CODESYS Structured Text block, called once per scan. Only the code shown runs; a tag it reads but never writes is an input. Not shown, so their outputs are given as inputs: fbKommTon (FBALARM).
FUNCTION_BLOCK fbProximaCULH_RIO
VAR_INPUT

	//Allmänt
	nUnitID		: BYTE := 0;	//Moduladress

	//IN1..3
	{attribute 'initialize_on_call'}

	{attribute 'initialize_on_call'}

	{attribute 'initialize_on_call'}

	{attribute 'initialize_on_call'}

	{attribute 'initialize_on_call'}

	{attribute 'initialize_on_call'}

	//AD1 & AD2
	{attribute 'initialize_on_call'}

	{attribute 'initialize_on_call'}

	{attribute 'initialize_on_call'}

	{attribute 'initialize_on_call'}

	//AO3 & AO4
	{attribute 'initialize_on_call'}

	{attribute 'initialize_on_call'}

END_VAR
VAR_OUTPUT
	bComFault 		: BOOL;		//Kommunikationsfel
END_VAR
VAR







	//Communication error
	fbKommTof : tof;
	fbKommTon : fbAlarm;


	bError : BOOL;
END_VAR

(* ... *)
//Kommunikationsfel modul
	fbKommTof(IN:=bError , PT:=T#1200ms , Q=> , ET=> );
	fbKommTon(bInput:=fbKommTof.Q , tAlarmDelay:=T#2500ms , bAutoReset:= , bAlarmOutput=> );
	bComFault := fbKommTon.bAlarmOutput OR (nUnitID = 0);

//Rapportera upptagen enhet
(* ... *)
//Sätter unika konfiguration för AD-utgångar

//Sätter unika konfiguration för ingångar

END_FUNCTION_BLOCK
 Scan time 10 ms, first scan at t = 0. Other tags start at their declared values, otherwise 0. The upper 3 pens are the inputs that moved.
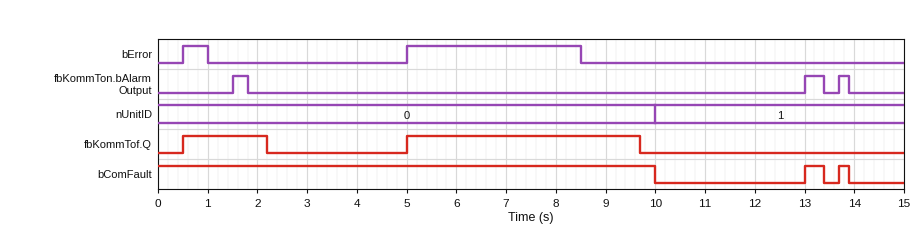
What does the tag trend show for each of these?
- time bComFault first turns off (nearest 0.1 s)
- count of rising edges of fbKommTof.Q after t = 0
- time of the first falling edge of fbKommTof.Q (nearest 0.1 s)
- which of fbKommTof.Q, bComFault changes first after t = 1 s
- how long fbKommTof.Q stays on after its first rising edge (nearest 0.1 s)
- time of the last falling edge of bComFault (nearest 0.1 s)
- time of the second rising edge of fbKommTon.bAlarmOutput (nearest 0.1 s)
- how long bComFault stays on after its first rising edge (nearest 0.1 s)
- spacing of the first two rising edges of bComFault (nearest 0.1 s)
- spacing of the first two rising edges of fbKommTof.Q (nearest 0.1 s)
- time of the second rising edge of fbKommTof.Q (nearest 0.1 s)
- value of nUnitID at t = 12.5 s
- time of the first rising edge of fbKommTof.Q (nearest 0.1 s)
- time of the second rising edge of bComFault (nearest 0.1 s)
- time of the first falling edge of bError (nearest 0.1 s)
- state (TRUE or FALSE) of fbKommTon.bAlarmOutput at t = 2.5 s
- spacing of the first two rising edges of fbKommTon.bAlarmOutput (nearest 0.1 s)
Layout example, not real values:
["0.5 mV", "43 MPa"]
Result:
["10.0 s", "2", "2.2 s", "fbKommTof.Q", "1.7 s", "13.9 s", "13.0 s", "0.4 s", "0.7 s", "4.5 s", "5.0 s", "1", "0.5 s", "13.7 s", "1.0 s", "FALSE", "11.5 s"]
